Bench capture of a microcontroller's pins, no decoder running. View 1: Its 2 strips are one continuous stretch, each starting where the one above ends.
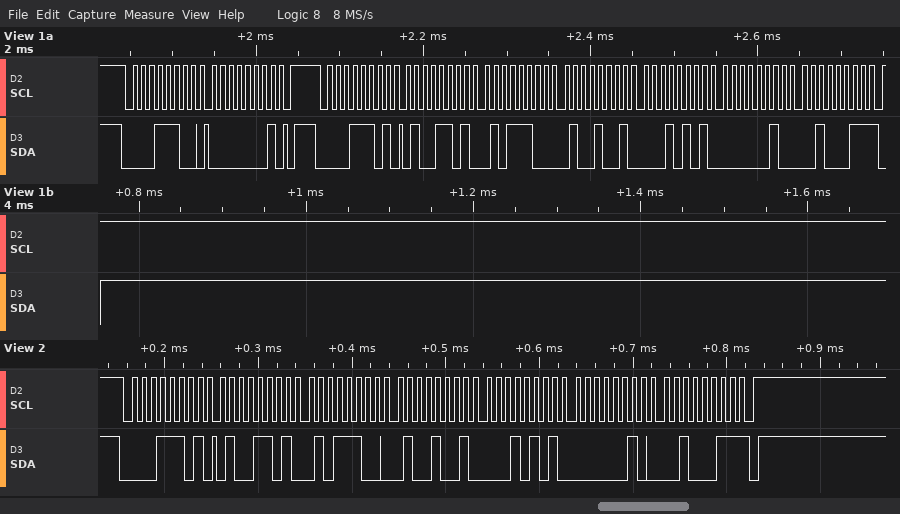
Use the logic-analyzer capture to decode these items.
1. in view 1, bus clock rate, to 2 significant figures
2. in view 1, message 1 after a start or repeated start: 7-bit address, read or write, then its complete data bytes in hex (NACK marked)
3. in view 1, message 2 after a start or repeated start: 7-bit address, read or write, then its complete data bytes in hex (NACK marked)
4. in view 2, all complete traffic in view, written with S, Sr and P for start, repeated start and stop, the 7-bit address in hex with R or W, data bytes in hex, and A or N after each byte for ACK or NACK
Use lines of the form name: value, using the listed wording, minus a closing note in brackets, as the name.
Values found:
in view 1, bus clock rate, to 2 significant figures: 100 kHz
in view 1, message 1 after a start or repeated start: 7-bit address, read or write, then its complete data bytes in hex: 0x0E write: 01
in view 1, message 2 after a start or repeated start: 7-bit address, read or write, then its complete data bytes in hex: 0x0E read: 4D 5C 49 15 02 23 NACK
in view 2, all complete traffic in view, written with S, Sr and P for start, repeated start and stop, the 7-bit address in hex with R or W, data bytes in hex, and A or N after each byte for ACK or NACK: S 0ER A 4D A 5C A 49 A 15 A 02 A 23 N P
